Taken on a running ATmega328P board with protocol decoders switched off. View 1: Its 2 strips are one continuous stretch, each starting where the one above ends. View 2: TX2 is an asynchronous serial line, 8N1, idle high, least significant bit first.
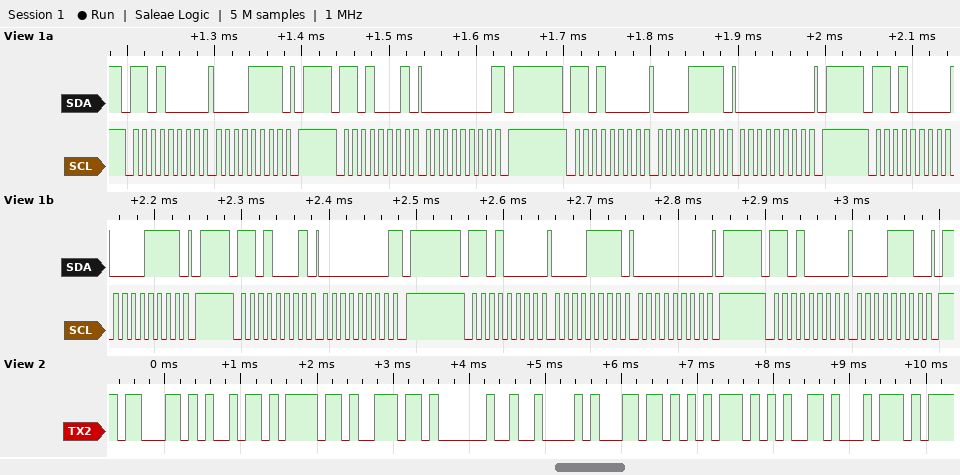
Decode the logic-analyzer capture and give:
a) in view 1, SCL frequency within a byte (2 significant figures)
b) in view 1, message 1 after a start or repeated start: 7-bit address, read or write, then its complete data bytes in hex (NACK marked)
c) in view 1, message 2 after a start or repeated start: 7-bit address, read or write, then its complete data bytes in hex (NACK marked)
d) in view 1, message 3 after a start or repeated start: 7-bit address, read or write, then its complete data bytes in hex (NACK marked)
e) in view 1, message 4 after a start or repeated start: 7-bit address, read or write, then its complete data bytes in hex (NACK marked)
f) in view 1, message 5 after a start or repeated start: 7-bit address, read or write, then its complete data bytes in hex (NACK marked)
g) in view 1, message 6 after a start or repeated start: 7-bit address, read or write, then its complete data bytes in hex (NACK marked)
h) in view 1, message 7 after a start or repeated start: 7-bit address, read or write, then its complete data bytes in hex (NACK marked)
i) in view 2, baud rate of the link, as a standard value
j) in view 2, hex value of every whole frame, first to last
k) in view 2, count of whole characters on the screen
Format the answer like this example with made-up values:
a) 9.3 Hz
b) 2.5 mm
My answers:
a) 100 kHz
b) 0x68 write: 0F
c) 0x68 read: 00 NACK
d) 0x68 write: 0F 00
e) 0x68 write: 0F
f) 0x68 read: 00 NACK
g) 0x68 write: 0F 00
h) 0x68 write: 0E
i) 9600 baud
j) 63 69 6F 6E 20 42 6C 75 65 74
k) 10
